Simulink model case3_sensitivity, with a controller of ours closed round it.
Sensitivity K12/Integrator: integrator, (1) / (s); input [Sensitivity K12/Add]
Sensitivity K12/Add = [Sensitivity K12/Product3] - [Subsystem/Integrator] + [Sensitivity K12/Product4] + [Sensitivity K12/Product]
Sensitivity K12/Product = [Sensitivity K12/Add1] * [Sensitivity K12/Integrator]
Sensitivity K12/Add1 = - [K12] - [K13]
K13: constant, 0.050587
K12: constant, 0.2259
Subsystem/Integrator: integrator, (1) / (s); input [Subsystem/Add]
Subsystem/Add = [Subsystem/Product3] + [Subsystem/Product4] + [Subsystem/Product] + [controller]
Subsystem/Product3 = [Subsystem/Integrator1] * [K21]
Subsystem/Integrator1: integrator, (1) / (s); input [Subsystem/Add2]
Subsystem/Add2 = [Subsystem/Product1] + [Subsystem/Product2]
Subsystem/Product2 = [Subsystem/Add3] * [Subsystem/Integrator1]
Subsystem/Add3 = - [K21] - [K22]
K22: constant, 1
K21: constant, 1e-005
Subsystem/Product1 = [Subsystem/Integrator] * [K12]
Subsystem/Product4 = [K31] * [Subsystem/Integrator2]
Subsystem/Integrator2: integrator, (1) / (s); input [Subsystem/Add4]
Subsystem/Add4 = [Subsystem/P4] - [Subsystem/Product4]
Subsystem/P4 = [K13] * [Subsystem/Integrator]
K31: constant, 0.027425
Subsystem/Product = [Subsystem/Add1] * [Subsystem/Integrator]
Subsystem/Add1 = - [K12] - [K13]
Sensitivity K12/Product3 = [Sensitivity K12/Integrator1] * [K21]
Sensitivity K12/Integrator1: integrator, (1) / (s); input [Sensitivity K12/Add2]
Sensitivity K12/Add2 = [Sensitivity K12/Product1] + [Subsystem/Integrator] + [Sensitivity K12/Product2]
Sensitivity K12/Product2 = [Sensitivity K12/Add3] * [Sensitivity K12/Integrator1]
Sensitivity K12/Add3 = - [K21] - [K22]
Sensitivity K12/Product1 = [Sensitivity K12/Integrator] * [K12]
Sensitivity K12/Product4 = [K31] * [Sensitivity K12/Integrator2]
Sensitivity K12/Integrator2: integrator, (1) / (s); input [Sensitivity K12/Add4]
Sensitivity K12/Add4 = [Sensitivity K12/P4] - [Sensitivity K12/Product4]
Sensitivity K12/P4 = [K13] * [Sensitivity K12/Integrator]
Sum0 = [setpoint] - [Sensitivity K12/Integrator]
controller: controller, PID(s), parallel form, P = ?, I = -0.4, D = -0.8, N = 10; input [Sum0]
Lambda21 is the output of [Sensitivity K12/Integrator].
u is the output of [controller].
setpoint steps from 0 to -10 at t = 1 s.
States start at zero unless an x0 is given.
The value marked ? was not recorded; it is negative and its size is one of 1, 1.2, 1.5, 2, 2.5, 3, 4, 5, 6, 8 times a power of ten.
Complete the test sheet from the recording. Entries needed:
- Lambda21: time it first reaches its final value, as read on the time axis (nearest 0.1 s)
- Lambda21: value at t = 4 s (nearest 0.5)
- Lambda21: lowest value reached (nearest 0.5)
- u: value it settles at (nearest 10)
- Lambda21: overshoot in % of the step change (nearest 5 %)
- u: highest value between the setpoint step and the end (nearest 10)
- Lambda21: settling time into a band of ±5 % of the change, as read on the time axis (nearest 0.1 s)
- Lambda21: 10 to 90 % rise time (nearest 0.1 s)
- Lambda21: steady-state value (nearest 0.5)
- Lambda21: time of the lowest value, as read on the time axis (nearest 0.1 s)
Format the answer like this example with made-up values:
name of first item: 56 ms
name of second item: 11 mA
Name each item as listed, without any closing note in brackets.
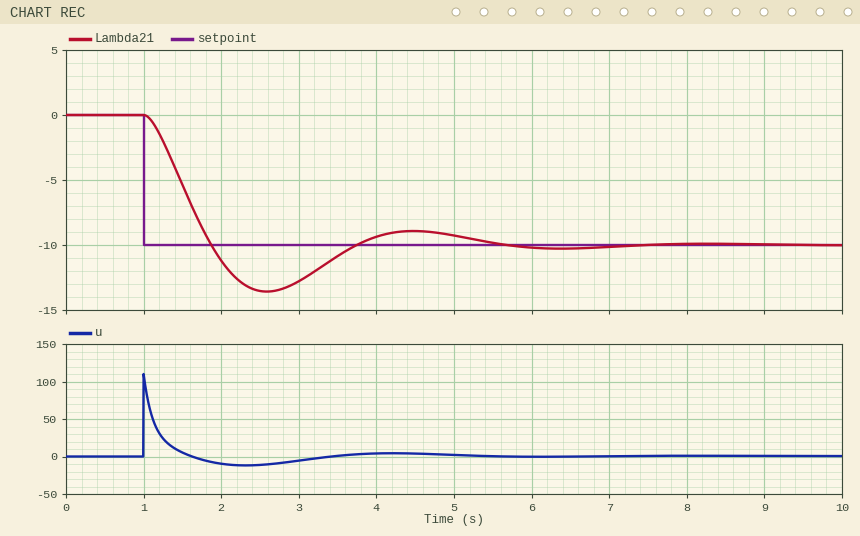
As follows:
Lambda21: time it first reaches its final value, as read on the time axis: 1.9 s
Lambda21: value at t = 4 s: -9.5
Lambda21: lowest value reached: -13.5
u: value it settles at: 0
Lambda21: overshoot in % of the step change: 35 %
u: highest value between the setpoint step and the end: 110
Lambda21: settling time into a band of ±5 % of the change, as read on the time axis: 5.2 s
Lambda21: 10 to 90 % rise time: 0.6 s
Lambda21: steady-state value: -10.0
Lambda21: time of the lowest value, as read on the time axis: 2.6 s
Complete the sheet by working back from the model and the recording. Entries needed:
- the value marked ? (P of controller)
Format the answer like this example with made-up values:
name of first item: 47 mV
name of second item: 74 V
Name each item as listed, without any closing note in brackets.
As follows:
the value marked ?: -3
